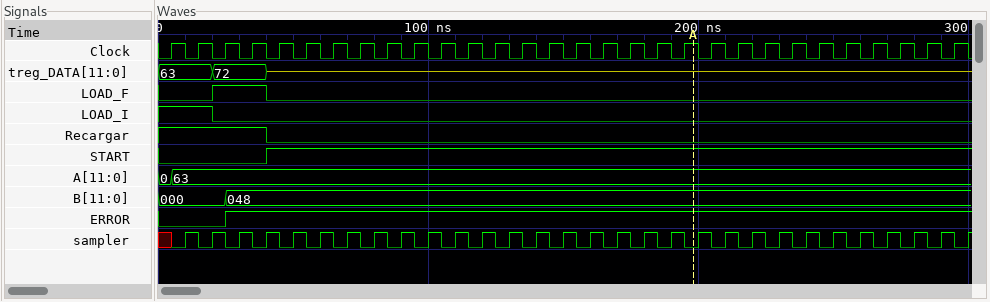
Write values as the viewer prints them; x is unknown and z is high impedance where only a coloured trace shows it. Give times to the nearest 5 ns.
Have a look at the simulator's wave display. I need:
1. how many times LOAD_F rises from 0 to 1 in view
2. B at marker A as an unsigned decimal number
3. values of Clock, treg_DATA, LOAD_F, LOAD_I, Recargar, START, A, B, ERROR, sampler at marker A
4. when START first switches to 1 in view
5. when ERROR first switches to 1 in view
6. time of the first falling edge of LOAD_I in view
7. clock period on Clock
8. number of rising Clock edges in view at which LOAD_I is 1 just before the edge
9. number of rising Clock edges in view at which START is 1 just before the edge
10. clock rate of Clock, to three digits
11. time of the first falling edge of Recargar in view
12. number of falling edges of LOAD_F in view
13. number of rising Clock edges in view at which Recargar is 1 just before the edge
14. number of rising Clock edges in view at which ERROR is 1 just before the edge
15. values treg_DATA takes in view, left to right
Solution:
1
72
Clock=1, treg_DATA=z, LOAD_F=0, LOAD_I=0, Recargar=0, START=1, A=63, B=048, ERROR=1, sampler=0
40 ns
25 ns
20 ns
10 ns
2
26
100 MHz
40 ns
1
4
27
63, 72, z
